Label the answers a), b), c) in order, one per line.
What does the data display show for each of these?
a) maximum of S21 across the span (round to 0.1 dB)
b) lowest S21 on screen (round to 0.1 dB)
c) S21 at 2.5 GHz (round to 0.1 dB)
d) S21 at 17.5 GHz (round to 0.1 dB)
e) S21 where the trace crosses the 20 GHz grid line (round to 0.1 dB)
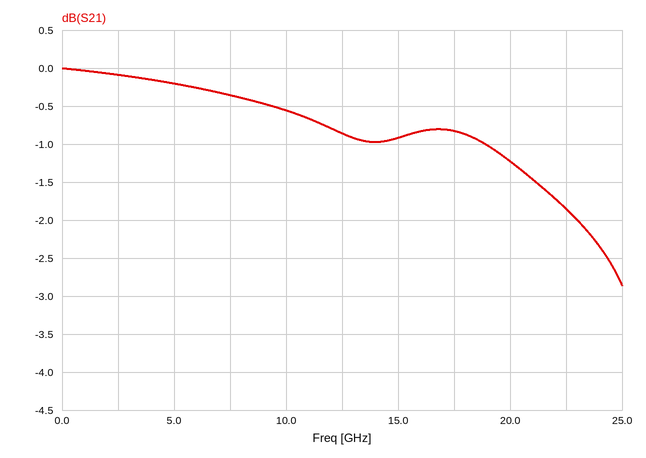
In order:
a) 0.0 dB
b) -2.9 dB
c) -0.1 dB
d) -0.8 dB
e) -1.2 dB
